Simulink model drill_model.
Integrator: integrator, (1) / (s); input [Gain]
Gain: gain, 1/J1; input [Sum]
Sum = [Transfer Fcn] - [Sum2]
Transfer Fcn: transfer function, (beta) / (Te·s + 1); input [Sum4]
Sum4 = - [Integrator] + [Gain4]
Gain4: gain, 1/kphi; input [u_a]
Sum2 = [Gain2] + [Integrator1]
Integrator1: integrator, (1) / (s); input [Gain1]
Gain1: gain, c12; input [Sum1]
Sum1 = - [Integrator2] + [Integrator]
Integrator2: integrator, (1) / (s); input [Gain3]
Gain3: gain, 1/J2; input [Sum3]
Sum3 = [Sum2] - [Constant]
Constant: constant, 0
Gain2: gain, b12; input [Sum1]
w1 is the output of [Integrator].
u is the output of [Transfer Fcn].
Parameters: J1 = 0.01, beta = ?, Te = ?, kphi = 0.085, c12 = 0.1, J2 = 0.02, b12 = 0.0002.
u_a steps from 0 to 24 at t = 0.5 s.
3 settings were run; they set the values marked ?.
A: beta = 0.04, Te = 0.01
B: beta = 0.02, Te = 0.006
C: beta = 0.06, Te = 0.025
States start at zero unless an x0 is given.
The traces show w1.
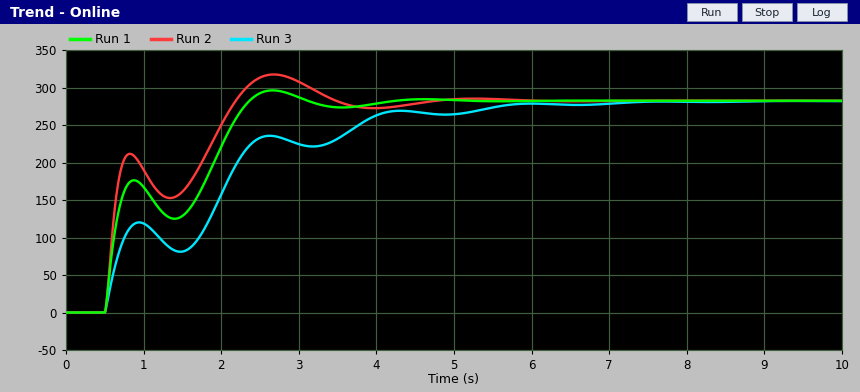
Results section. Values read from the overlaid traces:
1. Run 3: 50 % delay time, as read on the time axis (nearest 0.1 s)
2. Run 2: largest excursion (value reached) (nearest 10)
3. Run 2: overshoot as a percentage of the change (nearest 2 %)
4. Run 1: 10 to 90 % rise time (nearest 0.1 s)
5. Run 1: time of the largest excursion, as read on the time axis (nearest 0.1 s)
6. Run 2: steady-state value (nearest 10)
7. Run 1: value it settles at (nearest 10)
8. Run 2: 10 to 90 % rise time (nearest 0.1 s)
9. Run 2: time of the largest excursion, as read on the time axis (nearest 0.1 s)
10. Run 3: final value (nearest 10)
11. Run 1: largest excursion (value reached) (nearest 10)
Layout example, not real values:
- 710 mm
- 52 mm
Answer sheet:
- 1.9 s
- 320
- 12 %
- 1.6 s
- 2.7 s
- 280
- 280
- 1.5 s
- 2.7 s
- 280
- 300
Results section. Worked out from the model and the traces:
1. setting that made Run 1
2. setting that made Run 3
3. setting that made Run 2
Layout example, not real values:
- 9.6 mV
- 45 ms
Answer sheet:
- A
- B
- C
